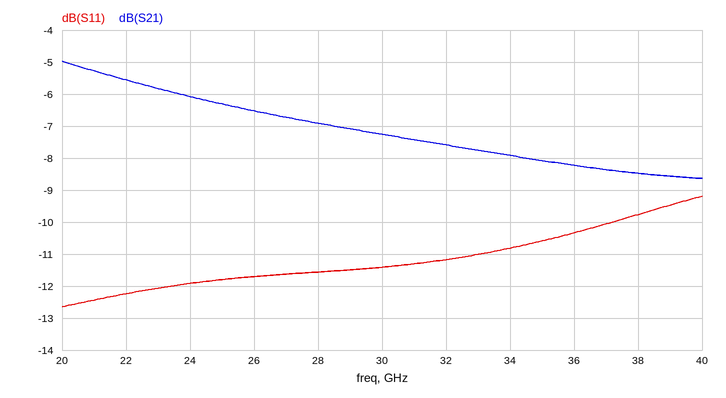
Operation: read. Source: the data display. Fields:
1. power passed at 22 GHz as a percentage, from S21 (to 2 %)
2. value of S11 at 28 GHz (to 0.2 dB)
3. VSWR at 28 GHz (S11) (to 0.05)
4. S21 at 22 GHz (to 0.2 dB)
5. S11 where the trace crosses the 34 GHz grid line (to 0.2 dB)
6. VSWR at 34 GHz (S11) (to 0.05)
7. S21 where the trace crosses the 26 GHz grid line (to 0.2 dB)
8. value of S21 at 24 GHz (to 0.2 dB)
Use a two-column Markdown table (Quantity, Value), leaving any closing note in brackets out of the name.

| Quantity | Value |
|---|---|
| power passed at 22 GHz as a percentage, from S21 | 28 % |
| value of S11 at 28 GHz | -11.6 dB |
| VSWR at 28 GHz (S11) | 1.70 |
| S21 at 22 GHz | -5.6 dB |
| S11 where the trace crosses the 34 GHz grid line | -10.8 dB |
| VSWR at 34 GHz (S11) | 1.80 |
| S21 where the trace crosses the 26 GHz grid line | -6.6 dB |
| value of S21 at 24 GHz | -6.0 dB |
